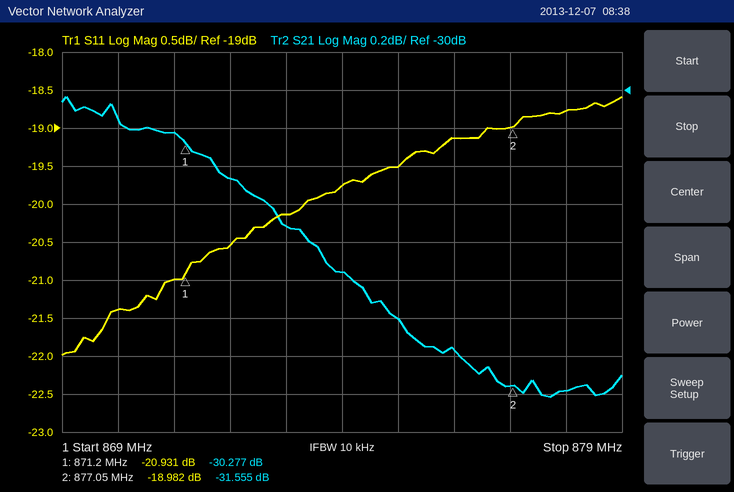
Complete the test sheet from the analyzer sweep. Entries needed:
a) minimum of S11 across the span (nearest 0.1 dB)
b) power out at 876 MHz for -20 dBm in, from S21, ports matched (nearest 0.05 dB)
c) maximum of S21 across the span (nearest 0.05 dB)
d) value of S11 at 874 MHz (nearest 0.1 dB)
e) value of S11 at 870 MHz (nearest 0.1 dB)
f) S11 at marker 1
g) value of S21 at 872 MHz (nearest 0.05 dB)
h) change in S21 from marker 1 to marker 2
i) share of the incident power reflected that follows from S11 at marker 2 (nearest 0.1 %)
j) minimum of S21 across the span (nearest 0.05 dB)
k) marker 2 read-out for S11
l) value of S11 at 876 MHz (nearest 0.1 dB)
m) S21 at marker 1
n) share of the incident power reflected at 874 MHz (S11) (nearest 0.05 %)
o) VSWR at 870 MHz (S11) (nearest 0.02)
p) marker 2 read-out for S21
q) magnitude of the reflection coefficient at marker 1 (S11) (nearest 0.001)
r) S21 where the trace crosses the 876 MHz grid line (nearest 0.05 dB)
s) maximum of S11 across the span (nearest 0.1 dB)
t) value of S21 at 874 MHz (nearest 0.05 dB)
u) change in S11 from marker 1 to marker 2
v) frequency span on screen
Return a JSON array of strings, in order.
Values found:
["-22.0 dB", "-51.35 dBm", "-30.05 dB", "-19.8 dB", "-21.4 dB", "-20.931 dB", "-30.45 dB", "-1.278 dB", "1.3 %", "-31.60 dB", "-18.982 dB", "-19.1 dB", "-30.277 dB", "1.05 %", "1.18", "-31.555 dB", "0.090", "-31.35 dB", "-18.6 dB", "-30.95 dB", "1.949 dB", "10 MHz"]
